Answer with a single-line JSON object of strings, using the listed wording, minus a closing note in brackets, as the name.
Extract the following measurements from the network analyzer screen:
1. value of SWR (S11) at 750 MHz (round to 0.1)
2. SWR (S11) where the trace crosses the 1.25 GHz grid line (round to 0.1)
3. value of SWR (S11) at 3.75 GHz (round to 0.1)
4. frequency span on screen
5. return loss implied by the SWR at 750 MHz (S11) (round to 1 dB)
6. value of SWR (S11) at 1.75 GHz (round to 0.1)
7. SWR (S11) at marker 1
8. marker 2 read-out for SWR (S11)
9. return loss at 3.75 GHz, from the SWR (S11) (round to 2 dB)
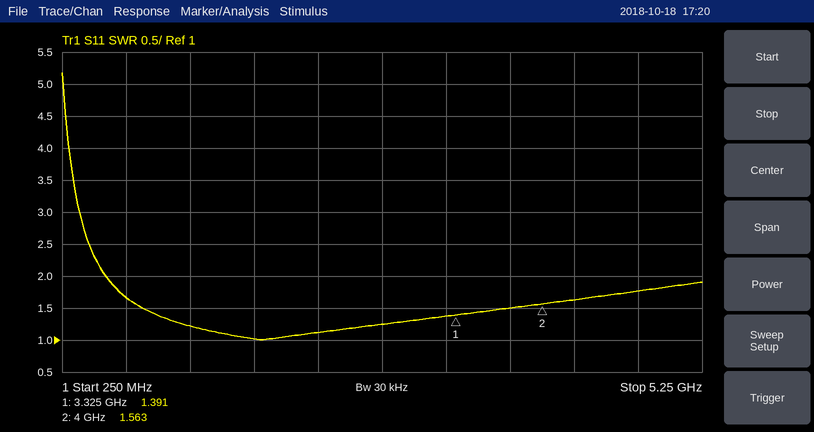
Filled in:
{"value of SWR (S11) at 750 MHz": "1.7", "SWR (S11) where the trace crosses the 1.25 GHz grid line": "1.2", "value of SWR (S11) at 3.75 GHz": "1.5", "frequency span on screen": "5 GHz", "return loss implied by the SWR at 750 MHz (S11)": "12 dB", "value of SWR (S11) at 1.75 GHz": "1.0", "SWR (S11) at marker 1": "1.391", "marker 2 read-out for SWR": "1.563", "return loss at 3.75 GHz, from the SWR (S11)": "14 dB"}
